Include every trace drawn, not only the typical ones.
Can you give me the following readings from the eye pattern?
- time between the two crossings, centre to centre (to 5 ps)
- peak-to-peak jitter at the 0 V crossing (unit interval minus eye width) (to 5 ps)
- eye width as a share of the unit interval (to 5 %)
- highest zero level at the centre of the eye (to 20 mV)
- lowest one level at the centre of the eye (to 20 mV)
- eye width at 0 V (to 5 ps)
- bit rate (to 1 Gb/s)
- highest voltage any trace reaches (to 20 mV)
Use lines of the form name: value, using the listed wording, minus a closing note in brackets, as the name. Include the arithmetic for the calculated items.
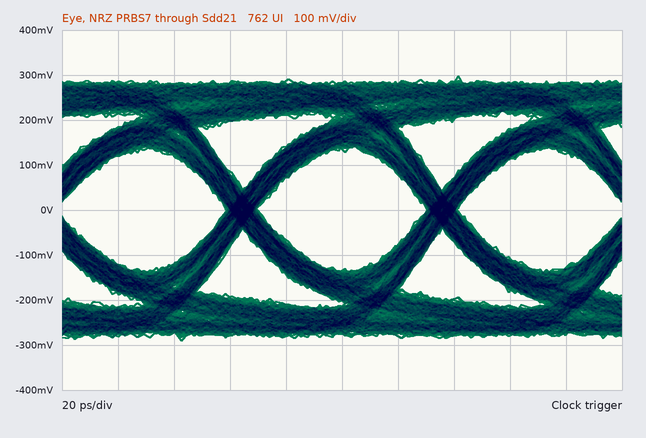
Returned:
time between the two crossings, centre to centre: 70 ps
peak-to-peak jitter at the 0 V crossing (unit interval minus eye width): 10 ps
eye width as a share of the unit interval: 60 ps / 70 ps ≈ 85.7 %, so 85 % to the nearest 5 %
highest zero level at the centre of the eye: -140 mV
lowest one level at the centre of the eye: 140 mV
eye width at 0 V: 60 ps
bit rate: 14 Gb/s
highest voltage any trace reaches: 300 mV
